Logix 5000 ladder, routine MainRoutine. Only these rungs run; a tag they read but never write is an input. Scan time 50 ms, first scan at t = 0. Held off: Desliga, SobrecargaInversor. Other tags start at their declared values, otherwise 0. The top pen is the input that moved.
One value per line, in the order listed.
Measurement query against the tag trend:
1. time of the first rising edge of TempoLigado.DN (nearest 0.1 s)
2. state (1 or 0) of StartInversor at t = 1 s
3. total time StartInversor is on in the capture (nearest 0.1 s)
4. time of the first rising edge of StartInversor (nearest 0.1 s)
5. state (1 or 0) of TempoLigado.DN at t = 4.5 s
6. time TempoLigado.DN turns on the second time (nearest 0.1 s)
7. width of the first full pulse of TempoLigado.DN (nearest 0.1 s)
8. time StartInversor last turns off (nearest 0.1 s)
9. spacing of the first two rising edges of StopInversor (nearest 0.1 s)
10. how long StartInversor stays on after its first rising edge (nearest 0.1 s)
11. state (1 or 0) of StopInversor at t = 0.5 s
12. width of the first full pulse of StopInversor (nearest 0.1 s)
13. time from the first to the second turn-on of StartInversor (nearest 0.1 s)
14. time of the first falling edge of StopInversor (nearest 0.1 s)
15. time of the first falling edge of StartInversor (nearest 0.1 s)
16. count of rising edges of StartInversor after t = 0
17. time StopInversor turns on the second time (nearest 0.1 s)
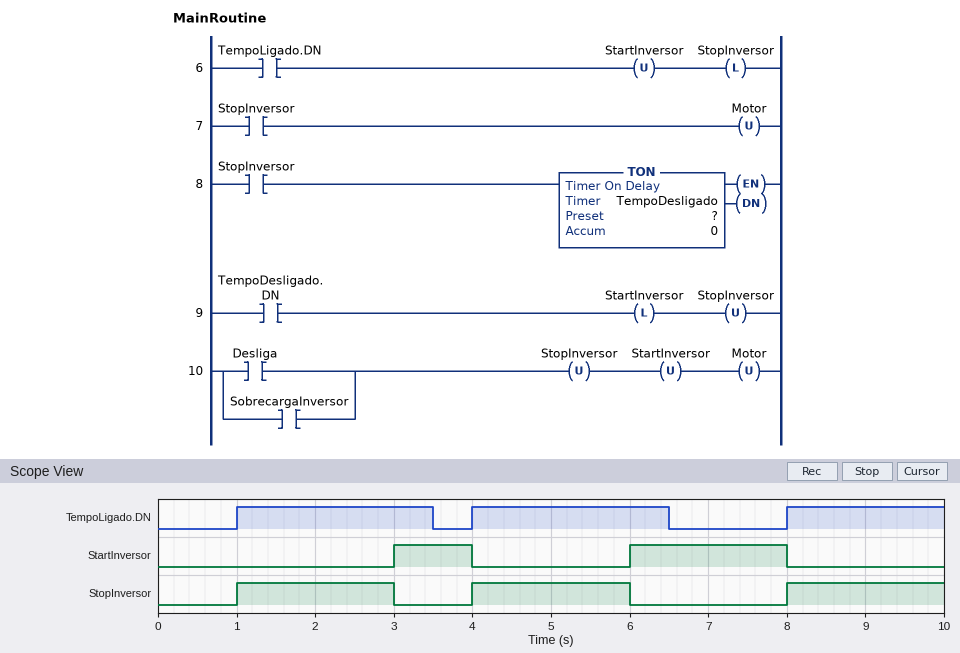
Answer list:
1.0 s
0
3.0 s
3.0 s
1
4.0 s
2.5 s
8.0 s
3.0 s
1.0 s
0
2.0 s
3.0 s
3.0 s
4.0 s
2
4.0 s
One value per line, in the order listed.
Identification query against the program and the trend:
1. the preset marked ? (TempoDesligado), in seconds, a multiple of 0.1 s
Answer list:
2.0 s
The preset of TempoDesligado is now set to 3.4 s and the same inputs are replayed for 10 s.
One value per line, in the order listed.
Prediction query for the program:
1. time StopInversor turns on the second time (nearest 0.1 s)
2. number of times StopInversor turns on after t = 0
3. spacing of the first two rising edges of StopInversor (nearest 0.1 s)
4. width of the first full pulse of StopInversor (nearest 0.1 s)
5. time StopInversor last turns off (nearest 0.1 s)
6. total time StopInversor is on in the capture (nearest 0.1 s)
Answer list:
8.0 s
2
7.0 s
3.4 s
4.4 s
5.4 s
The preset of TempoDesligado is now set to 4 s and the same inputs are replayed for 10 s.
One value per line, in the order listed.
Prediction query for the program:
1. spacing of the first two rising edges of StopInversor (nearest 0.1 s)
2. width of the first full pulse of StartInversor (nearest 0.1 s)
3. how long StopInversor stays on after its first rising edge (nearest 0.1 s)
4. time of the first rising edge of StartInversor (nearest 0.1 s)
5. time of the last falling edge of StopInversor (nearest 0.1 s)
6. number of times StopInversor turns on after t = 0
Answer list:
7.0 s
3.0 s
4.0 s
5.0 s
5.0 s
2
